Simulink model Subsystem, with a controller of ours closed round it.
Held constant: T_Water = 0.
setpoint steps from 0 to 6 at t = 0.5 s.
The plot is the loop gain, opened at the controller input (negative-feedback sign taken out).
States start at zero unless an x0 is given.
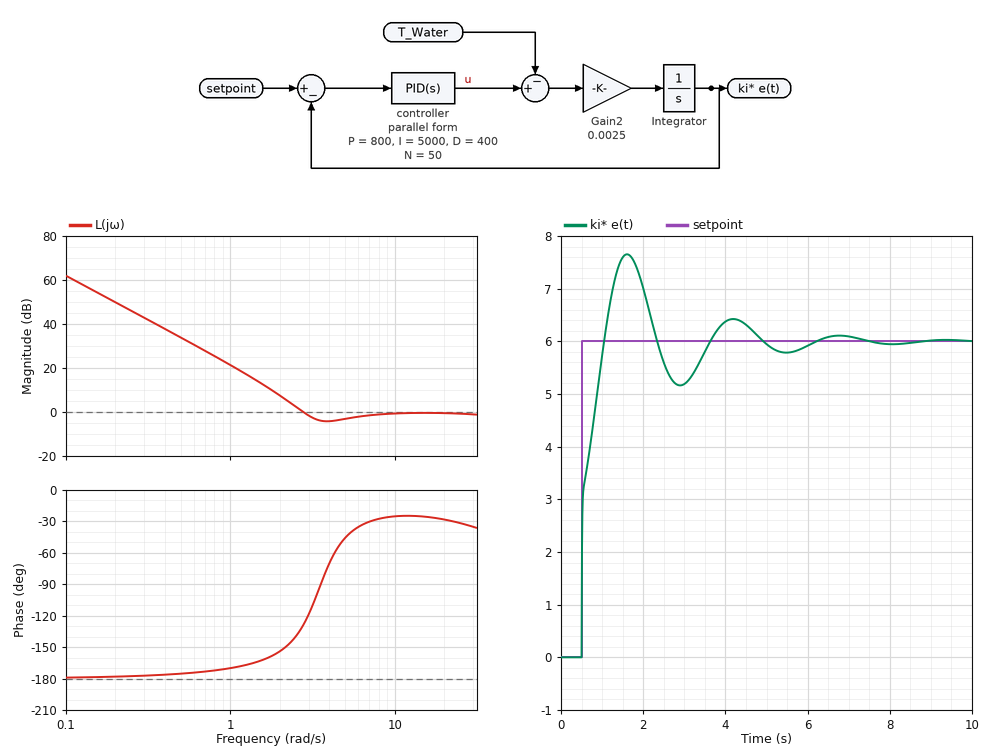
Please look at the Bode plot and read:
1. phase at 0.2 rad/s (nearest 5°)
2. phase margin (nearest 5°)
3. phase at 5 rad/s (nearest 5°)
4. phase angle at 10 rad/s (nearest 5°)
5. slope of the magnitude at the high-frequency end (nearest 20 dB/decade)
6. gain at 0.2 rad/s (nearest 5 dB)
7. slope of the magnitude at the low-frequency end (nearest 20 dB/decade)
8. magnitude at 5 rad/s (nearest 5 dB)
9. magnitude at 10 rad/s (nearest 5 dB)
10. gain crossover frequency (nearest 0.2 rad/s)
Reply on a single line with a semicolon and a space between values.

-180°; 50°; -45°; -25°; 0 dB/decade; 50 dB; -40 dB/decade; -5 dB; 0 dB; 2.8 rad/s
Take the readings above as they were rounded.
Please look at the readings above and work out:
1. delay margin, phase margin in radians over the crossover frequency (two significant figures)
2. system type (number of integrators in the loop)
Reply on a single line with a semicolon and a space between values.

0.31 s; 2
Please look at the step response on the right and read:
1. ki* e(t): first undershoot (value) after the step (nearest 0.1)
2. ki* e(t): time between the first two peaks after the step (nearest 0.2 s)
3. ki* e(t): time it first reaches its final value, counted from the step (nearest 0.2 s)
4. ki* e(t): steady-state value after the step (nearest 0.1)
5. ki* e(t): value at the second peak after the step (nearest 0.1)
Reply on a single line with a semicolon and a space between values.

5.2; 2.6 s; 0.6 s; 6.0; 6.4
